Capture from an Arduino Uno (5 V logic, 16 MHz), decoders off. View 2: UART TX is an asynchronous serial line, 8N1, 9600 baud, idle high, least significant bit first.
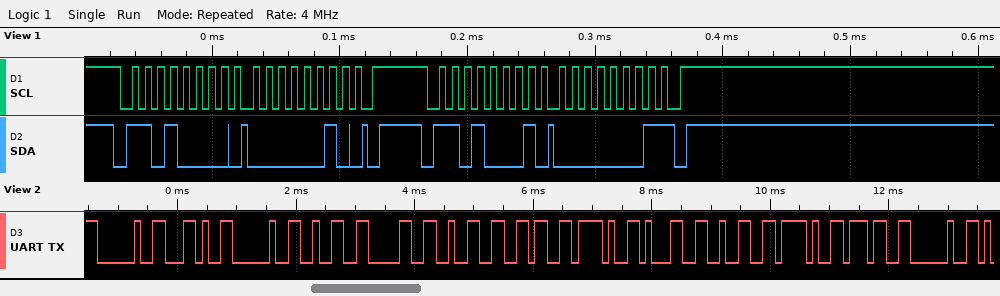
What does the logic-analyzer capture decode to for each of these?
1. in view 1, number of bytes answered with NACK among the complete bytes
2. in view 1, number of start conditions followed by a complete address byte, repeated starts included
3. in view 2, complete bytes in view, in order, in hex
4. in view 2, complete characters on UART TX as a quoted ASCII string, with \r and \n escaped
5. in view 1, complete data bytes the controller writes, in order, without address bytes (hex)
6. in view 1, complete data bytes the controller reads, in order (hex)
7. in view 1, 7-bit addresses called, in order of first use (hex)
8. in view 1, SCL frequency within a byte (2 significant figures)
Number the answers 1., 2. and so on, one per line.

1. 1
2. 2
3. 0x20 0x2C 0x20 0x32 0x30 0x32 0x36 0x2F 0x31 0x32 0x2F 0x37 0x20
4. " , 2026/12/7 "
5. 02
6. 01
7. 0x68
8. 100 kHz
